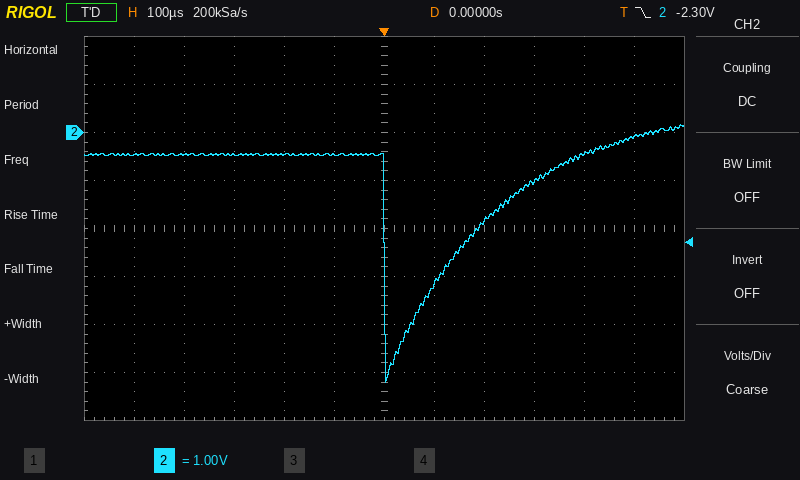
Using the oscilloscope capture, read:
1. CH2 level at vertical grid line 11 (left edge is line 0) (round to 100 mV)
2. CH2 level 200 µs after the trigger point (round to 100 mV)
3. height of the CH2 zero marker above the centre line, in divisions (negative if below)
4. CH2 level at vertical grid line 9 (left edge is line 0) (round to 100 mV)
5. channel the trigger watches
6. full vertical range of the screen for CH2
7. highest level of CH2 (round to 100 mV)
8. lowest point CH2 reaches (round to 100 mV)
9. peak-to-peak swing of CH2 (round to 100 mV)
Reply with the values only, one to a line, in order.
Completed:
-100 mV
-1.8 V
+2.0 div
-1.0 V
CH2
8 V
200 mV
-5.2 V
5.4 V
